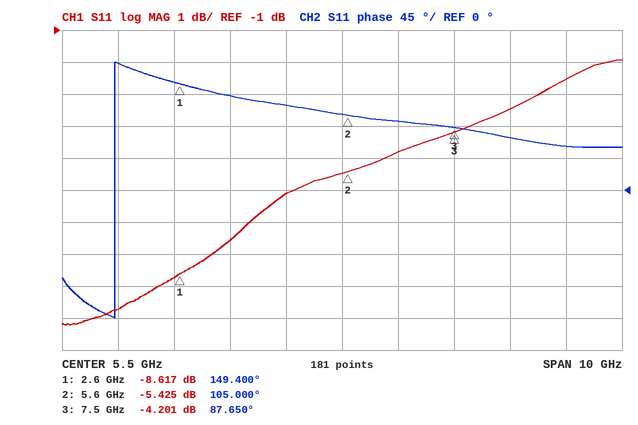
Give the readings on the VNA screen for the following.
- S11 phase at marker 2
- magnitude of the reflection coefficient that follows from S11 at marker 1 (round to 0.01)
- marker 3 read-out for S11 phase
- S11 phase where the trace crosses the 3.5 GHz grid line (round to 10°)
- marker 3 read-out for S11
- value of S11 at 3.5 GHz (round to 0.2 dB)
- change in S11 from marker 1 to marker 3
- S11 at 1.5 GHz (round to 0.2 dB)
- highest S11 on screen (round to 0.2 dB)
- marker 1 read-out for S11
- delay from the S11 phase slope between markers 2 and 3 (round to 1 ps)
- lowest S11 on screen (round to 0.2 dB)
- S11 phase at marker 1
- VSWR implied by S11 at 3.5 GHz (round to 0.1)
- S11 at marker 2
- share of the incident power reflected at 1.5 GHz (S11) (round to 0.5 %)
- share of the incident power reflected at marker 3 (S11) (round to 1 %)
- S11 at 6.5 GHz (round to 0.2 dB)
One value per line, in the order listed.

105.000°
0.37
87.650°
130°
-4.201 dB
-7.6 dB
4.416 dB
-9.8 dB
-2.0 dB
-8.617 dB
25 ps
-10.2 dB
149.400°
2.4
-5.425 dB
10.5 %
38 %
-4.8 dB
